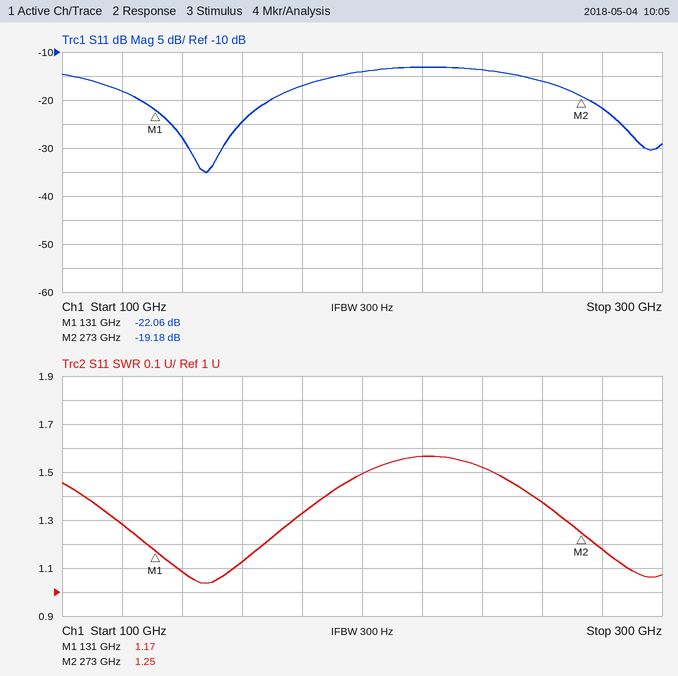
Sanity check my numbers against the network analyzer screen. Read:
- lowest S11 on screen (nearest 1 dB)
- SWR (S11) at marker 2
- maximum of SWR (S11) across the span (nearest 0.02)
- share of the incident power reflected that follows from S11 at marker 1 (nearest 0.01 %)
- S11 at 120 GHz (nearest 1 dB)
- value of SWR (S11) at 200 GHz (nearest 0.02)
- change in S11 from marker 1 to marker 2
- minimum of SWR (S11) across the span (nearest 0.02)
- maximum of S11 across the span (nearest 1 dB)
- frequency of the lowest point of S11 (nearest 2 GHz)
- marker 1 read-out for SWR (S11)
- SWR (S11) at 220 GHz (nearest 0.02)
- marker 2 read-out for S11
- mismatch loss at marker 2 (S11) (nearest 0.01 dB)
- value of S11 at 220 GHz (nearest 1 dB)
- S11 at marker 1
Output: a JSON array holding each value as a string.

["-35 dB", "1.25", "1.56", "0.62 %", "-18 dB", "1.50", "2.88 dB", "1.04", "-13 dB", "148 GHz", "1.17", "1.56", "-19.18 dB", "0.05 dB", "-13 dB", "-22.06 dB"]
